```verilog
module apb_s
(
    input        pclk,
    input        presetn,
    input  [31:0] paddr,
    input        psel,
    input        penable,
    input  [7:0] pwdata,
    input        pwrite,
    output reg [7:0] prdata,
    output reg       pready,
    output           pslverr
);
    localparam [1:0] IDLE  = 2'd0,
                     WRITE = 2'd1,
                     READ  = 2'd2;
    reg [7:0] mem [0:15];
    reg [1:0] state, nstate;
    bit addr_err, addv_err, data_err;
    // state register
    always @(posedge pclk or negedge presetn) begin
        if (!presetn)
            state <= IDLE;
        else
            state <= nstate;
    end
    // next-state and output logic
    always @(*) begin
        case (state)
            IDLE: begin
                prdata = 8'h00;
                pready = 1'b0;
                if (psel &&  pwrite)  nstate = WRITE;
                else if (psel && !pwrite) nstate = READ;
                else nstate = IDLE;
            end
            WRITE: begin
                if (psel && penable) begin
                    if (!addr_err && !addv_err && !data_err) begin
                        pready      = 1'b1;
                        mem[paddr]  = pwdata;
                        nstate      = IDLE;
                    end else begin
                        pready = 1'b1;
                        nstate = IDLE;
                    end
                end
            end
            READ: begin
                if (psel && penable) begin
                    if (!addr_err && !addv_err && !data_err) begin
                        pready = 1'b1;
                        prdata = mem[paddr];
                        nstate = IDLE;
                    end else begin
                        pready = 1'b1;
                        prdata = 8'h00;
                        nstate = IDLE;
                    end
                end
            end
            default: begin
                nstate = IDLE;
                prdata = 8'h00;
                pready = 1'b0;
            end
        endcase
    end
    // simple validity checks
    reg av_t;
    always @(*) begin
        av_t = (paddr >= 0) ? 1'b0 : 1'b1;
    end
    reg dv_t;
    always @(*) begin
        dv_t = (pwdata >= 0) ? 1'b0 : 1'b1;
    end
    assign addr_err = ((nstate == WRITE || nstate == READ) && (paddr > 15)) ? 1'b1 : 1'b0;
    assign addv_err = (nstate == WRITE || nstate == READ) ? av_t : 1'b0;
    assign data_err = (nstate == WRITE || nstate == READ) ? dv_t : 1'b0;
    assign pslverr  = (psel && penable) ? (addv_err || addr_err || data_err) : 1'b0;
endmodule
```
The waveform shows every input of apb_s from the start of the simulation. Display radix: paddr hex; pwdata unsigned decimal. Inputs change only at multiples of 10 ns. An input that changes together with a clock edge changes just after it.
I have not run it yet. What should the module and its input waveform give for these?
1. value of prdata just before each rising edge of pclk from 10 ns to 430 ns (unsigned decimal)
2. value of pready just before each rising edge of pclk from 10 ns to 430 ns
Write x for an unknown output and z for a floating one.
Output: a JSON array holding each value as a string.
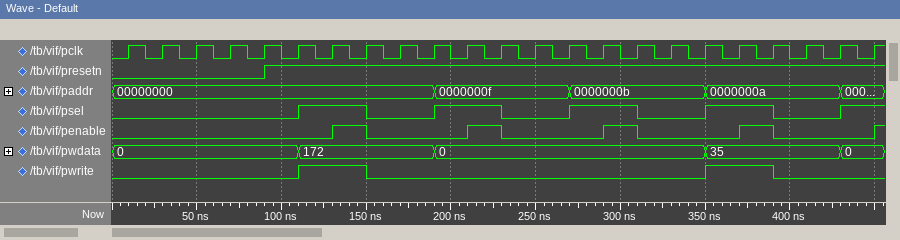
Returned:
["0, 0, 0, 0, 0, 0, 0, 0, 0, 0, 0, x, 0, 0, 0, x, 0, 0, 0, 0, 0, 0", "0 0 0 0 0 0 0 1 0 0 0 1 0 0 0 1 0 0 0 1 0 0"]
